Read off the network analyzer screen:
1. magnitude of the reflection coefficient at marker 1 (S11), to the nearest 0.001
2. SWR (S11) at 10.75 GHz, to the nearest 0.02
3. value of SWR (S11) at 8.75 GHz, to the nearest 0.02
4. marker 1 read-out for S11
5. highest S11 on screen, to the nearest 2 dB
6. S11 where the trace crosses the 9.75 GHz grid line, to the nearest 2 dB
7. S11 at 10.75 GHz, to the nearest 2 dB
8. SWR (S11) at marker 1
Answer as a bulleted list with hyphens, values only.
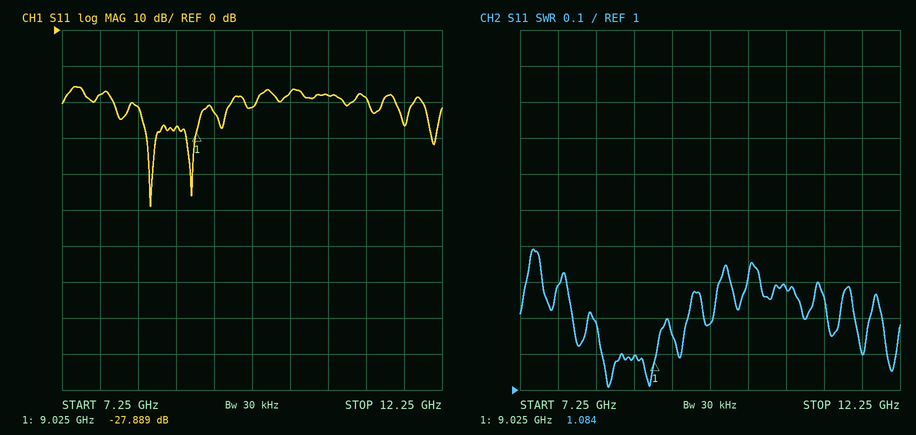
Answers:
- 0.040
- 1.28
- 1.10
- -27.889 dB
- -16 dB
- -22 dB
- -18 dB
- 1.084
